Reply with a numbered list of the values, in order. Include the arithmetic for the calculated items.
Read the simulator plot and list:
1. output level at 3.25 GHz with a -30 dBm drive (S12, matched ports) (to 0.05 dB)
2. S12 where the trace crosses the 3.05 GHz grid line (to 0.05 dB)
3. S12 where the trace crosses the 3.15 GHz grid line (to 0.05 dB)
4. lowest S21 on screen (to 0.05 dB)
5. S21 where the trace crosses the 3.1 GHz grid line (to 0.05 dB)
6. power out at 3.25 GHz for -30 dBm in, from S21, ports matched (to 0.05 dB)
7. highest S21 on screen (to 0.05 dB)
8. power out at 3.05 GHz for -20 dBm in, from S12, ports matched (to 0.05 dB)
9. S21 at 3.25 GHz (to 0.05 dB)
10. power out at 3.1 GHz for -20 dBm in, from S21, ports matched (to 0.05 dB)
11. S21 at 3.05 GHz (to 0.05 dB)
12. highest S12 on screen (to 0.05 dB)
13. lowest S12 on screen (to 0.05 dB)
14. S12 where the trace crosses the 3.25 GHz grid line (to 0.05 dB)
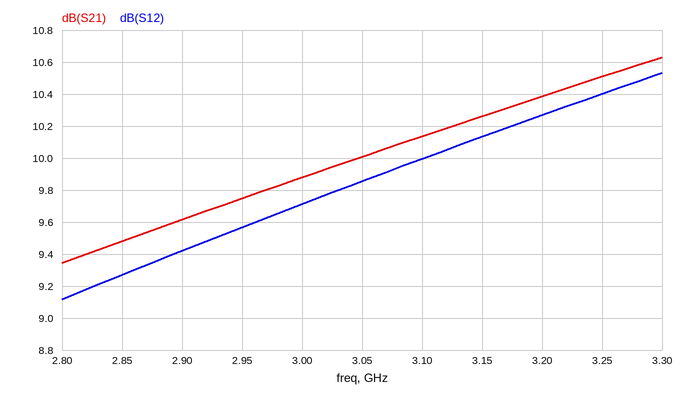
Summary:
1. -30 dBm + (10.40 dB) = -19.60 dBm
2. 9.85 dB
3. 10.15 dB
4. 9.35 dB
5. 10.15 dB
6. -30 dBm + (10.50 dB) = -19.50 dBm
7. 10.65 dB
8. -20 dBm + (9.85 dB) = -10.15 dBm
9. 10.50 dB
10. -20 dBm + (10.15 dB) = -9.85 dBm
11. 10.00 dB
12. 10.55 dB
13. 9.10 dB
14. 10.40 dB
